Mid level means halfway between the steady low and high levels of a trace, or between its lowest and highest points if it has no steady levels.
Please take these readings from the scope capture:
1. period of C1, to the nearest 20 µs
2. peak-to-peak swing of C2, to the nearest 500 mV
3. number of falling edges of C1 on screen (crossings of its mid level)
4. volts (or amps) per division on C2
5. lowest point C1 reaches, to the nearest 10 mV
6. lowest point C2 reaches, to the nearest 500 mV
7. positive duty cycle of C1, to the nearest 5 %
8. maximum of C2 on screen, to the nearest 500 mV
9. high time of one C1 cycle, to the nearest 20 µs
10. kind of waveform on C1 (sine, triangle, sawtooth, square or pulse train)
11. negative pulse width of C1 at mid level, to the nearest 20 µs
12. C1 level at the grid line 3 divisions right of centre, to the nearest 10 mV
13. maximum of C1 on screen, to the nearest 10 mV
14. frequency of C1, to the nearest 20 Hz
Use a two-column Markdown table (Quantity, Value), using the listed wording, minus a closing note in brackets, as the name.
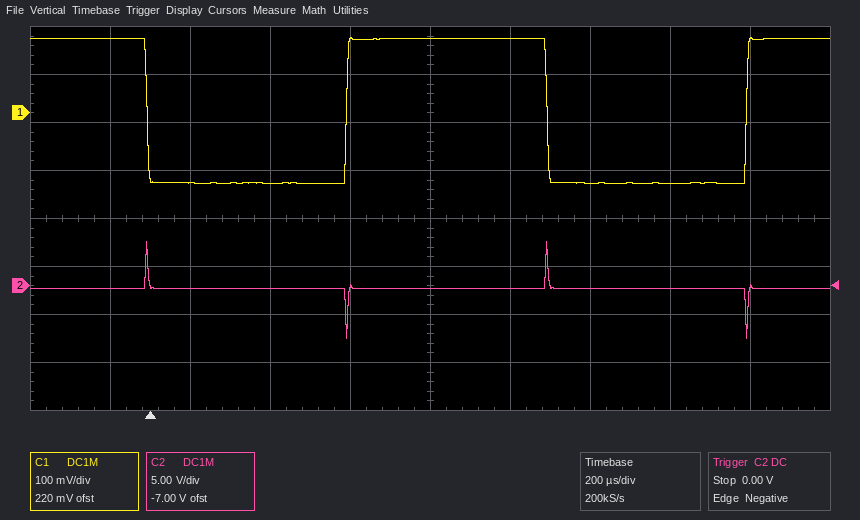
| Quantity | Value |
|---|---|
| period of C1, to the nearest 20 µs | 1.00 ms |
| peak-to-peak swing of C2, to the nearest 500 mV | 10.0 V |
| number of falling edges of C1 on screen | 2 |
| volts (or amps) per division on C2 | 5 V |
| lowest point C1 reaches, to the nearest 10 mV | -150 mV |
| lowest point C2 reaches, to the nearest 500 mV | -5.5 V |
| positive duty cycle of C1, to the nearest 5 % | 50 % |
| maximum of C2 on screen, to the nearest 500 mV | 4.5 V |
| high time of one C1 cycle, to the nearest 20 µs | 500 µs |
| kind of waveform on C1 | square |
| negative pulse width of C1 at mid level, to the nearest 20 µs | 500 µs |
| C1 level at the grid line 3 divisions right of centre, to the nearest 10 mV | -150 mV |
| maximum of C1 on screen, to the nearest 10 mV | 160 mV |
| frequency of C1, to the nearest 20 Hz | 1.00 kHz |
